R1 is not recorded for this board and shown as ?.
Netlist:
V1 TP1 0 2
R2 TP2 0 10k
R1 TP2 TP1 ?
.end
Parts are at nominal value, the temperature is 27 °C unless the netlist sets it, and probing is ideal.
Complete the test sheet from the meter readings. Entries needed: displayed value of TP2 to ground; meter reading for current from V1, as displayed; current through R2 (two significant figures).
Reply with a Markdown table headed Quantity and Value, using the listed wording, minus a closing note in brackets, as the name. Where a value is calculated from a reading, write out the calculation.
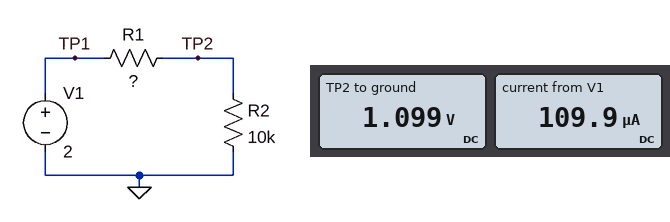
| Quantity | Value |
|---|---|
| displayed value of TP2 to ground | 1.099 V |
| meter reading for current from V1, as displayed | 109.9 µA |
| current through R2 | (1.099 V) / 10 kΩ = 110 µA |
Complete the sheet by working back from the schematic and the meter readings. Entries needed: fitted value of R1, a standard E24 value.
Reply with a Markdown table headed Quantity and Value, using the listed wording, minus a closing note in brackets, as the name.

| Quantity | Value |
|---|---|
| fitted value of R1, a standard E24 value | 8.2 kΩ |
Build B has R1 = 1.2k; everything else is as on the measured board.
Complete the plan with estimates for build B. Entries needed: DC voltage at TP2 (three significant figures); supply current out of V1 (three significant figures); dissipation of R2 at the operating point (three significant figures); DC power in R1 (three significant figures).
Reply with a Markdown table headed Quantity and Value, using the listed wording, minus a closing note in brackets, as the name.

| Quantity | Value |
|---|---|
| DC voltage at TP2 | 1.79 V |
| supply current out of V1 | 179 µA |
| dissipation of R2 at the operating point | 319 µW |
| DC power in R1 | 38.3 µW |
